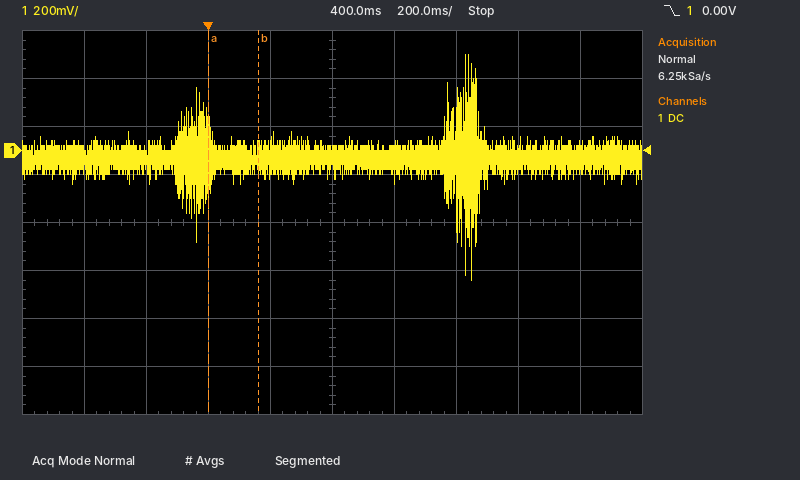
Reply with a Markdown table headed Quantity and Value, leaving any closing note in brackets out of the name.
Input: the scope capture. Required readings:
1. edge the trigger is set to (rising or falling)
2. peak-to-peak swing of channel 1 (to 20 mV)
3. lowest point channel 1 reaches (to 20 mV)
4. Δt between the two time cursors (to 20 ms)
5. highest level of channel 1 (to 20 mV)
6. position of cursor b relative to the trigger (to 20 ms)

| Quantity | Value |
|---|---|
| edge the trigger is set to | falling |
| peak-to-peak swing of channel 1 | 940 mV |
| lowest point channel 1 reaches | -540 mV |
| Δt between the two time cursors | 160 ms |
| highest level of channel 1 | 400 mV |
| position of cursor b relative to the trigger | +160 ms |
